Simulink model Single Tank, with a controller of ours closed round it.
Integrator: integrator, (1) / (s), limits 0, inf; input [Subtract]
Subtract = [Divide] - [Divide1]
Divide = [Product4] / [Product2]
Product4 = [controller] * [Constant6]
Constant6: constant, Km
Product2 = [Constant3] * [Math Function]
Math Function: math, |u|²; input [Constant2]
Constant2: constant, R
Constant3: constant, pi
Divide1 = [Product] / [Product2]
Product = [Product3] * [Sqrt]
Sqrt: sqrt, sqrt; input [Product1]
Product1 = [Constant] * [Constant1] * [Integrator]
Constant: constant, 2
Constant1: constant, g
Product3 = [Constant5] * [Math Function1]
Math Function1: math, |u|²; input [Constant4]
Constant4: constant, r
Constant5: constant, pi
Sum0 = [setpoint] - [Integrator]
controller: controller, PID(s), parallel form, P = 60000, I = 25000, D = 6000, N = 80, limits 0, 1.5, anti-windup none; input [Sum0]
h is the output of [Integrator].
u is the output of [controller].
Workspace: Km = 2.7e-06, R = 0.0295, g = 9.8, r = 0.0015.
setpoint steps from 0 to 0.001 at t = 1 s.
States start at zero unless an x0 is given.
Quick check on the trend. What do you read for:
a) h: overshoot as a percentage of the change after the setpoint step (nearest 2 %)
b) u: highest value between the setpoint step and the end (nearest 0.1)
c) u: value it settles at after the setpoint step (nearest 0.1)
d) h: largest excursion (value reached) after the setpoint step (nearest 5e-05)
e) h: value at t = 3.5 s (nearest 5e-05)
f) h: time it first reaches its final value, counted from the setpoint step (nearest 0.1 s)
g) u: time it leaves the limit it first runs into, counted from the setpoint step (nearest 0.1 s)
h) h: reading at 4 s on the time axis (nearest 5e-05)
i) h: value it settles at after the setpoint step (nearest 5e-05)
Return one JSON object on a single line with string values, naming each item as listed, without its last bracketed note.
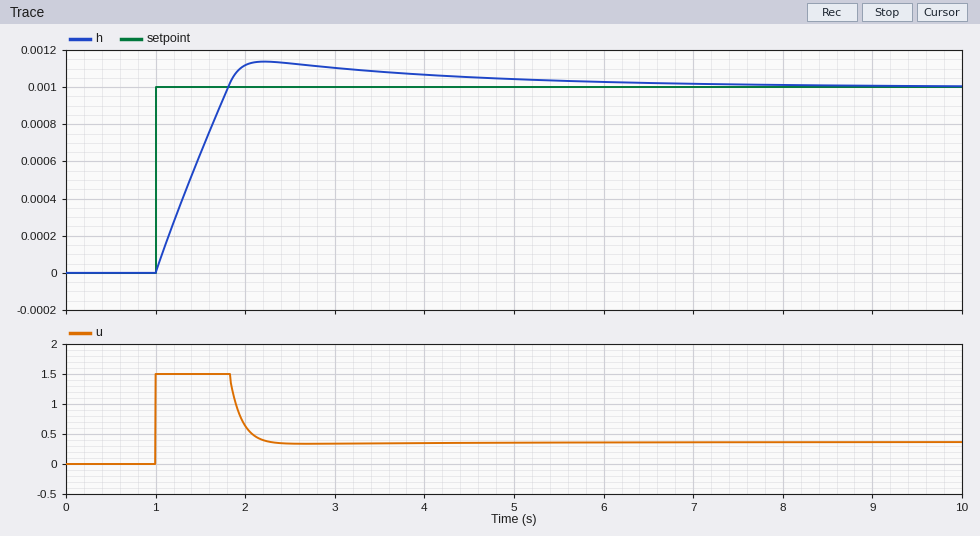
{"h: overshoot as a percentage of the change after the setpoint step": "14 %", "u: highest value between the setpoint step and the end": "1.5", "u: value it settles at after the setpoint step": "0.4", "h: largest excursion (value reached) after the setpoint step": "0.00115", "h: value at t = 3.5 s": "0.00110", "h: time it first reaches its final value, counted from the setpoint step": "0.8 s", "u: time it leaves the limit it first runs into, counted from the setpoint step": "0.8 s", "h: reading at 4 s on the time axis": "0.00105", "h: value it settles at after the setpoint step": "0.00100"}
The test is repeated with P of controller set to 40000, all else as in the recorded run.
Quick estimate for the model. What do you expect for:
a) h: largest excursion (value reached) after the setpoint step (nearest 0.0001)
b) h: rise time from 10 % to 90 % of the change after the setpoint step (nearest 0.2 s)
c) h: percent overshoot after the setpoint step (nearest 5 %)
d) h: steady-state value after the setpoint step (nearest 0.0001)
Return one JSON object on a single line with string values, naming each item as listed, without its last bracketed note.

{"h: largest excursion (value reached) after the setpoint step": "0.0012", "h: rise time from 10 % to 90 % of the change after the setpoint step": "0.6 s", "h: percent overshoot after the setpoint step": "20 %", "h: steady-state value after the setpoint step": "0.0010"}
